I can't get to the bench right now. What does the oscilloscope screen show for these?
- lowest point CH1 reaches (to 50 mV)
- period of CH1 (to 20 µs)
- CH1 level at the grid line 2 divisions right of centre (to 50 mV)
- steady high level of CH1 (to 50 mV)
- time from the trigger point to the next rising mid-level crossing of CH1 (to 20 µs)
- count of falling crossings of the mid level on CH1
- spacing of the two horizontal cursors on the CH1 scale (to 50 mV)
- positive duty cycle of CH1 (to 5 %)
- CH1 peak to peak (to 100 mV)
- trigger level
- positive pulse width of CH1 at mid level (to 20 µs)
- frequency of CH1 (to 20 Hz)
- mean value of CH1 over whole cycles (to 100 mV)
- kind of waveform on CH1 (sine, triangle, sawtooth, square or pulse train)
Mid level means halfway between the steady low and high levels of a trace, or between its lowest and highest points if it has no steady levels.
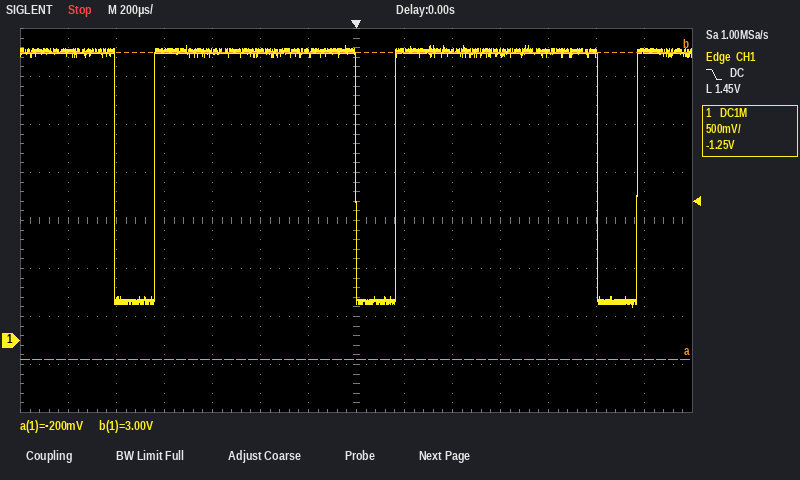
350 mV
1.00 ms
3.00 V
3.00 V
160 µs
3
3.20 V
85 %
2.70 V
1.45 V
840 µs
1.00 kHz
2.6 V
pulse train
